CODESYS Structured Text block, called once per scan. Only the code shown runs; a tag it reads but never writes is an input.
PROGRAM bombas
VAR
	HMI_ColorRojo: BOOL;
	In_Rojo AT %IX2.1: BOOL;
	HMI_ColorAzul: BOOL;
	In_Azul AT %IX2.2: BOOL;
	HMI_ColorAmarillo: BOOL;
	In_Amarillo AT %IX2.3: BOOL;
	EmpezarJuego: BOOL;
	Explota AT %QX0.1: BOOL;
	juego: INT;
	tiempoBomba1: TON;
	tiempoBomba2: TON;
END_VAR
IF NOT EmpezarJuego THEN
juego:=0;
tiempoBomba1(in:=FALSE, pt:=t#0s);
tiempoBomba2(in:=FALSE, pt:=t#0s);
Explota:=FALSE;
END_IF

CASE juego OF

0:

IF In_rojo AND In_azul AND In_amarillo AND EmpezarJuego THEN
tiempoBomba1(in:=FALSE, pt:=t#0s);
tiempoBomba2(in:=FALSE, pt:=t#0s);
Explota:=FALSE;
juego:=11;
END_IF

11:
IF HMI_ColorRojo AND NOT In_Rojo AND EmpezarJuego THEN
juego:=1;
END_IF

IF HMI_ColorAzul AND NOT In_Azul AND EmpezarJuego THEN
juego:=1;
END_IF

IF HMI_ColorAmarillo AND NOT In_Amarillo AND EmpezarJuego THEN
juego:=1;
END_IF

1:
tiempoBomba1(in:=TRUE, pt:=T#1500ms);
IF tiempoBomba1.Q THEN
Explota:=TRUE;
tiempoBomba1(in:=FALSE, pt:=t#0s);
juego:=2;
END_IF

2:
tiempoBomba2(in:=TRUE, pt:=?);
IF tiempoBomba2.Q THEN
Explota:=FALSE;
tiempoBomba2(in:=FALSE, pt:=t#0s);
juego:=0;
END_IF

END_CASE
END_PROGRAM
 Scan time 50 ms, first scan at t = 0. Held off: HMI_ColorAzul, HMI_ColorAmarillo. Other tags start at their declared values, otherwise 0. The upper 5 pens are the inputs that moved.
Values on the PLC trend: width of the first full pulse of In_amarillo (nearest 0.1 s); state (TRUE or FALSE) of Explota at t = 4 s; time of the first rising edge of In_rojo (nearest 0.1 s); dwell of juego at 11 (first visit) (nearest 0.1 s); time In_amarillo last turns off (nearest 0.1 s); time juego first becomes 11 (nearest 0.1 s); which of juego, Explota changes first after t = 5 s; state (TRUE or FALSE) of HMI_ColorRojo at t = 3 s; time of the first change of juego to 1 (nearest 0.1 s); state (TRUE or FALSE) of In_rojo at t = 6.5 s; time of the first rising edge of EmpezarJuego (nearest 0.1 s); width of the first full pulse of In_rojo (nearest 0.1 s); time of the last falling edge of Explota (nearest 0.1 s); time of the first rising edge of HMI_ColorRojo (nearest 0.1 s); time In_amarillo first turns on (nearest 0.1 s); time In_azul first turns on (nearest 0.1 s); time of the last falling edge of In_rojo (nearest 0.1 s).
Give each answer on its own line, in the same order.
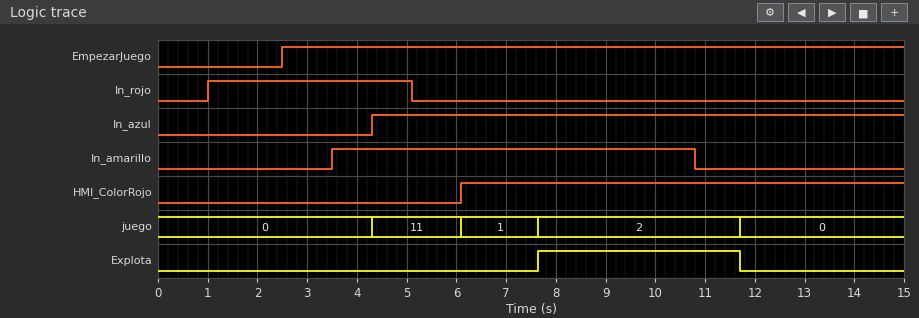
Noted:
7.3 s
FALSE
1.0 s
1.8 s
10.8 s
4.3 s
juego
FALSE
6.1 s
FALSE
2.5 s
4.1 s
11.7 s
6.1 s
3.5 s
4.3 s
5.1 s
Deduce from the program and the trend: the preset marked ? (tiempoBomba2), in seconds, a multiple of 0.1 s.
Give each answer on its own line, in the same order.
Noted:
4.0 s
